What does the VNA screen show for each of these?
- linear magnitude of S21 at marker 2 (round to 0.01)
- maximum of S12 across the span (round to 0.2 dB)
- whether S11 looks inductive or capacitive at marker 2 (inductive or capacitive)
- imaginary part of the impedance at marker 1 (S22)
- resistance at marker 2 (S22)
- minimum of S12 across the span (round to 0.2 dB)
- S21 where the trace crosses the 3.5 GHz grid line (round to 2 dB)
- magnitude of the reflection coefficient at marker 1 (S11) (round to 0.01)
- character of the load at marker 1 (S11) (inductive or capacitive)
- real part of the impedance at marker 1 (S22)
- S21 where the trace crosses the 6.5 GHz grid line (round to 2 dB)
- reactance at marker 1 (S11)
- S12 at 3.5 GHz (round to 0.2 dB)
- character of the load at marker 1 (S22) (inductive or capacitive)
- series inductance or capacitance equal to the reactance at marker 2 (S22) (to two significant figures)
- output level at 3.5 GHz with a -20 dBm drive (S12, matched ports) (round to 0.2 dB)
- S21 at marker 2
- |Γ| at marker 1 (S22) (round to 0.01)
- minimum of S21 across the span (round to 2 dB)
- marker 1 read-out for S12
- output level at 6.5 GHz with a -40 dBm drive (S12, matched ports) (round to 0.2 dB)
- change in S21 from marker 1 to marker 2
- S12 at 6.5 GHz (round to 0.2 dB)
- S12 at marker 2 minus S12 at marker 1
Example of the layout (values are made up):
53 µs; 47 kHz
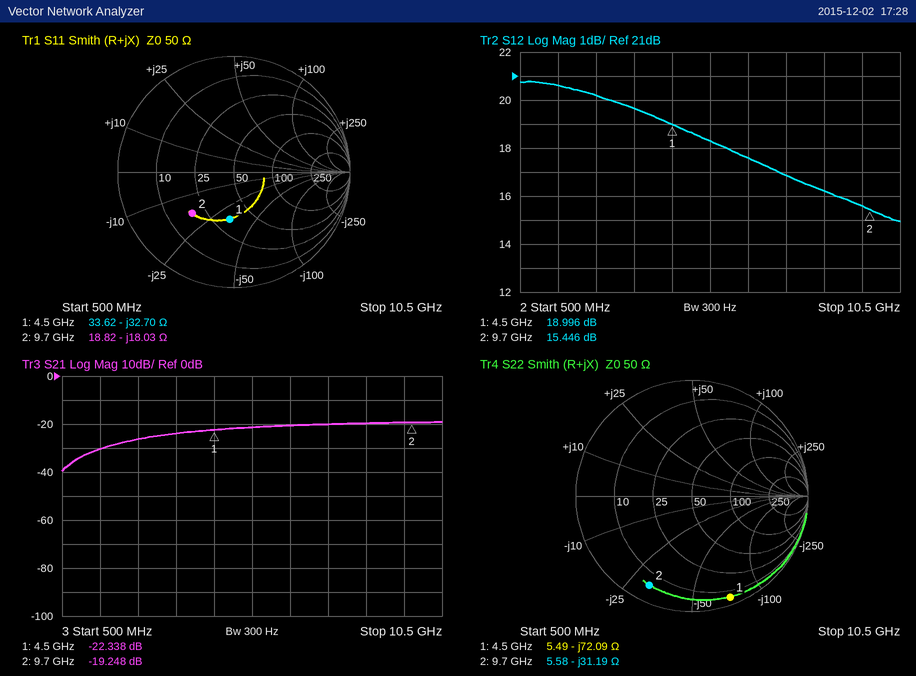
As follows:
0.11; 20.8 dB; capacitive; -72.09 Ω; 5.58 Ω; 15.0 dB; -24 dB; 0.41; capacitive; 5.49 Ω; -20 dB; -32.70 Ω; 19.6 dB; capacitive; 530 fF; -0.4 dBm; -19.248 dB; 0.93; -40 dB; 18.996 dB; -22.4 dBm; 3.090 dB; 17.6 dB; -3.550 dB
